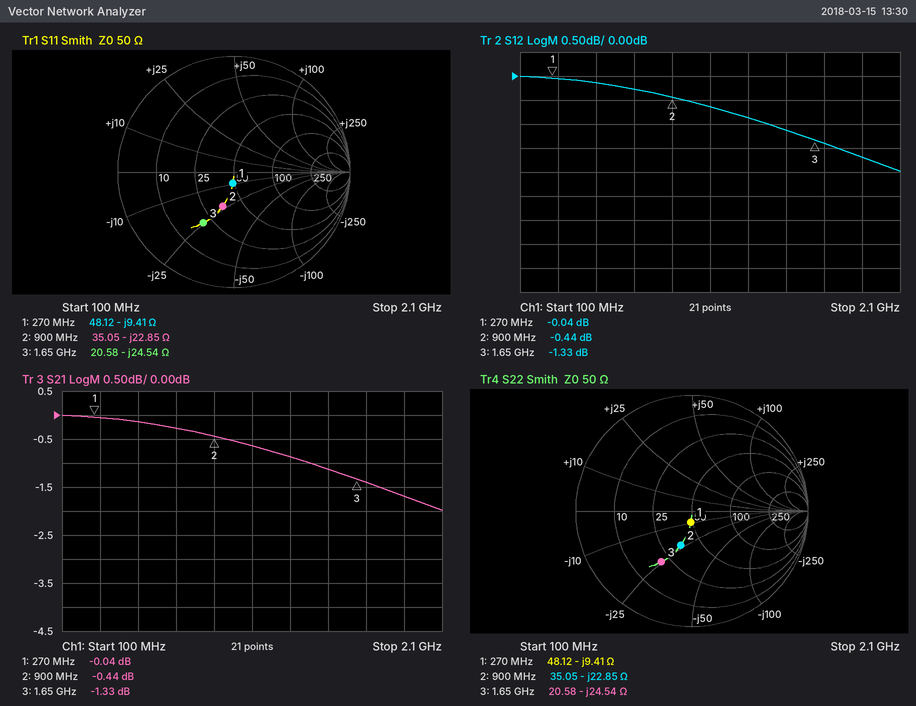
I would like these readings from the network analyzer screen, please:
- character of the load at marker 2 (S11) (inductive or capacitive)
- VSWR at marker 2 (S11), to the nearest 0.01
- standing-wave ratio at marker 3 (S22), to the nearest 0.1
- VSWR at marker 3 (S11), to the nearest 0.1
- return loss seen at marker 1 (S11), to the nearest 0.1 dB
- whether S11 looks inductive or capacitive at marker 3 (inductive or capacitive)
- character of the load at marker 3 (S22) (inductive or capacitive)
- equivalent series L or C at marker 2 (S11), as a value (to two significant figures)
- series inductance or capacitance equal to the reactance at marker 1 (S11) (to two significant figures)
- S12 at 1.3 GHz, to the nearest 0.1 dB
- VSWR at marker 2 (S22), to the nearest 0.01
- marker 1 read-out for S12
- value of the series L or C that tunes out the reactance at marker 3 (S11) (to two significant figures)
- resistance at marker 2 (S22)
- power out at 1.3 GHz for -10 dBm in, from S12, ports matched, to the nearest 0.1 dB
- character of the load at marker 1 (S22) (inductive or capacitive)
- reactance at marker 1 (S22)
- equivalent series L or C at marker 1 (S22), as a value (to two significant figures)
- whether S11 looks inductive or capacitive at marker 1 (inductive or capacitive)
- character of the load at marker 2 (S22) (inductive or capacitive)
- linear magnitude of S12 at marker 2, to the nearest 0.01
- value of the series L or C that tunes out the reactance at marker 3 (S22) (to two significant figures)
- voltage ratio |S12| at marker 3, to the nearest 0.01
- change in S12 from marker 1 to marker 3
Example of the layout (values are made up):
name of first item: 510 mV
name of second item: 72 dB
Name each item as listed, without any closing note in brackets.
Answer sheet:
character of the load at marker 2 (S11): capacitive
VSWR at marker 2 (S11), to the nearest 0.01: 1.90
standing-wave ratio at marker 3 (S22), to the nearest 0.1: 3.1
VSWR at marker 3 (S11), to the nearest 0.1: 3.1
return loss seen at marker 1 (S11), to the nearest 0.1 dB: 20.2 dB
whether S11 looks inductive or capacitive at marker 3: capacitive
character of the load at marker 3 (S22): capacitive
equivalent series L or C at marker 2 (S11), as a value: 7.7 pF
series inductance or capacitance equal to the reactance at marker 1 (S11): 63 pF
S12 at 1.3 GHz, to the nearest 0.1 dB: -0.9 dB
VSWR at marker 2 (S22), to the nearest 0.01: 1.90
marker 1 read-out for S12: -0.04 dB
value of the series L or C that tunes out the reactance at marker 3 (S11): 2.4 nH
resistance at marker 2: 35.05 Ω
power out at 1.3 GHz for -10 dBm in, from S12, ports matched, to the nearest 0.1 dB: -10.9 dBm
character of the load at marker 1 (S22): capacitive
reactance at marker 1: -9.41 Ω
equivalent series L or C at marker 1 (S22), as a value: 63 pF
whether S11 looks inductive or capacitive at marker 1: capacitive
character of the load at marker 2 (S22): capacitive
linear magnitude of S12 at marker 2, to the nearest 0.01: 0.95
value of the series L or C that tunes out the reactance at marker 3 (S22): 2.4 nH
voltage ratio |S12| at marker 3, to the nearest 0.01: 0.86
change in S12 from marker 1 to marker 3: -1.29 dB
